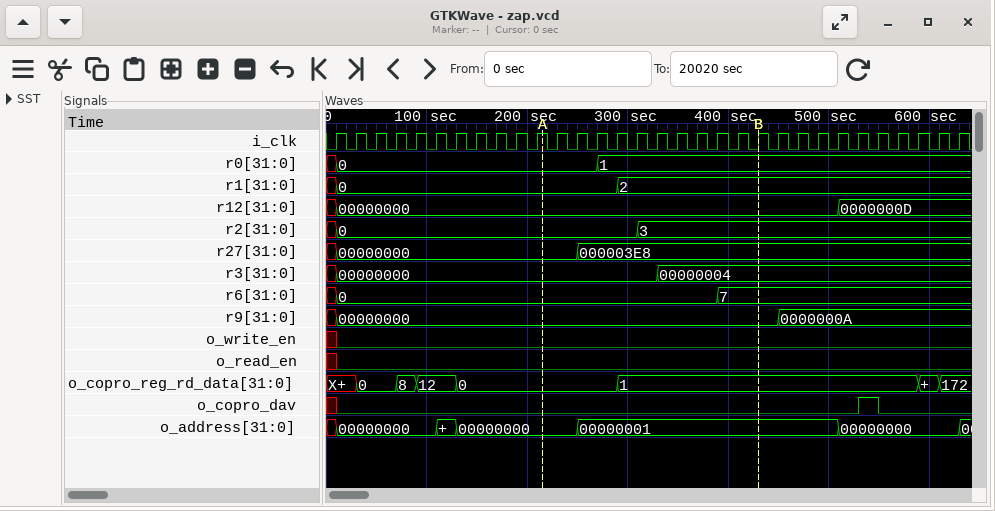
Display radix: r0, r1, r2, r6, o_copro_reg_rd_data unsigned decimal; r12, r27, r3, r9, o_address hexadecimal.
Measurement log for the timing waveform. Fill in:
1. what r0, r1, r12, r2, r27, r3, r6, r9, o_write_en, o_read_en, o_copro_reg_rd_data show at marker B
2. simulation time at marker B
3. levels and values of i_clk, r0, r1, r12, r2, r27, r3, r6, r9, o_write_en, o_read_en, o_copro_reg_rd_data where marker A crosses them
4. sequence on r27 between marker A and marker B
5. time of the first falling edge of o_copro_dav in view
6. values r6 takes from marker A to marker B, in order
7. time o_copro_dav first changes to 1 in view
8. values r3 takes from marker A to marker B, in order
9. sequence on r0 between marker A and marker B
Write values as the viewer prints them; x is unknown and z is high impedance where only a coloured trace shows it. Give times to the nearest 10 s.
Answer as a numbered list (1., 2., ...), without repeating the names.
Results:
1. r0=1, r1=2, r12=00000000, r2=3, r27=000003E8, r3=00000004, r6=7, r9=00000000, o_write_en=0, o_read_en=0, o_copro_reg_rd_data=1
2. 430 s
3. i_clk=1, r0=0, r1=0, r12=00000000, r2=0, r27=00000000, r3=00000000, r6=0, r9=00000000, o_write_en=0, o_read_en=0, o_copro_reg_rd_data=0
4. 00000000, 000003E8
5. 550 s
6. 0, 7
7. 530 s
8. 00000000, 00000004
9. 0, 1
